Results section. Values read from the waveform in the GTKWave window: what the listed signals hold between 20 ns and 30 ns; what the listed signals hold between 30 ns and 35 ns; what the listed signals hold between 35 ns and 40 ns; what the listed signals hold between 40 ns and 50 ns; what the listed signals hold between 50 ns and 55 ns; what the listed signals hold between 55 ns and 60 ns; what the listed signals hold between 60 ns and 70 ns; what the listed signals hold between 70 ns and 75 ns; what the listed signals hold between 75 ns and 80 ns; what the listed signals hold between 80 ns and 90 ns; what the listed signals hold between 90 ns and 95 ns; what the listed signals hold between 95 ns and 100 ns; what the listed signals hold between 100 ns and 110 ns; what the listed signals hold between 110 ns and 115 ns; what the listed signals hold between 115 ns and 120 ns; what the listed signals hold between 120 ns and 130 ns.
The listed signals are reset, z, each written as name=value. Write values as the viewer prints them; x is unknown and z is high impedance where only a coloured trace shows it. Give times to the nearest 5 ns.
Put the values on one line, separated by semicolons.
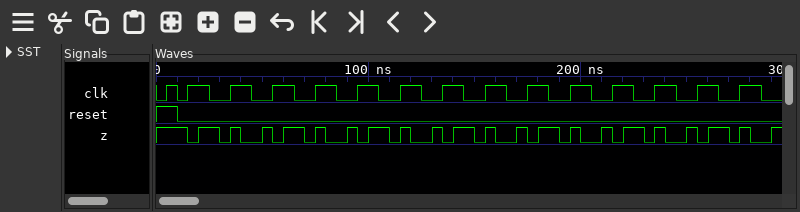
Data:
reset=0, z=1; reset=0, z=0; reset=0, z=1; reset=0, z=0; reset=0, z=1; reset=0, z=0; reset=0, z=1; reset=0, z=0; reset=0, z=1; reset=0, z=0; reset=0, z=1; reset=0, z=0; reset=0, z=1; reset=0, z=0; reset=0, z=1; reset=0, z=0
